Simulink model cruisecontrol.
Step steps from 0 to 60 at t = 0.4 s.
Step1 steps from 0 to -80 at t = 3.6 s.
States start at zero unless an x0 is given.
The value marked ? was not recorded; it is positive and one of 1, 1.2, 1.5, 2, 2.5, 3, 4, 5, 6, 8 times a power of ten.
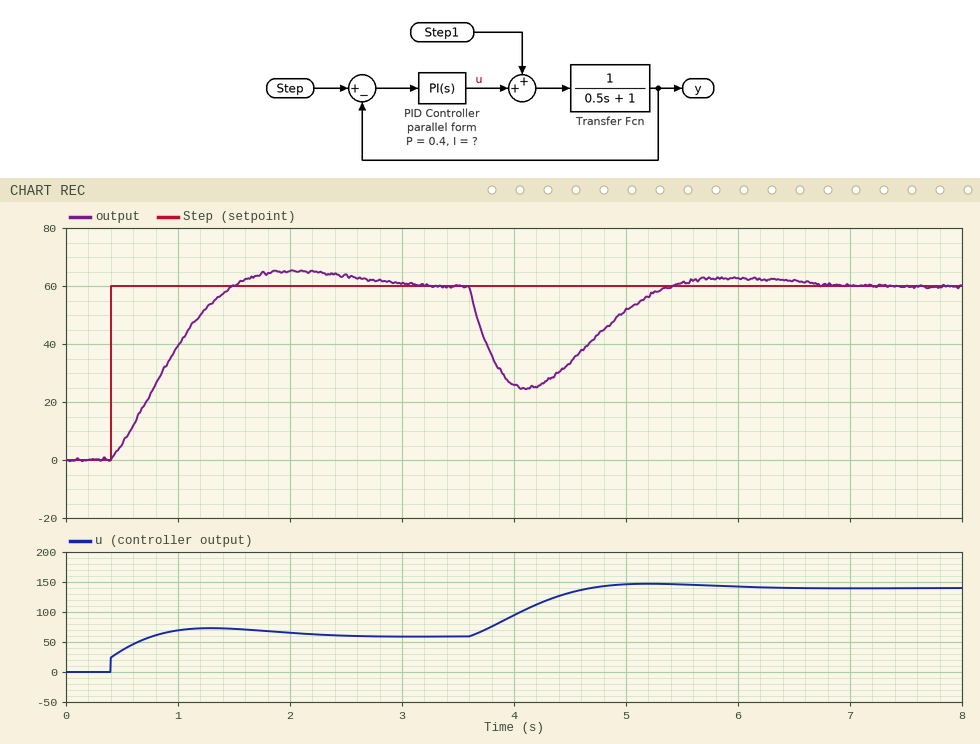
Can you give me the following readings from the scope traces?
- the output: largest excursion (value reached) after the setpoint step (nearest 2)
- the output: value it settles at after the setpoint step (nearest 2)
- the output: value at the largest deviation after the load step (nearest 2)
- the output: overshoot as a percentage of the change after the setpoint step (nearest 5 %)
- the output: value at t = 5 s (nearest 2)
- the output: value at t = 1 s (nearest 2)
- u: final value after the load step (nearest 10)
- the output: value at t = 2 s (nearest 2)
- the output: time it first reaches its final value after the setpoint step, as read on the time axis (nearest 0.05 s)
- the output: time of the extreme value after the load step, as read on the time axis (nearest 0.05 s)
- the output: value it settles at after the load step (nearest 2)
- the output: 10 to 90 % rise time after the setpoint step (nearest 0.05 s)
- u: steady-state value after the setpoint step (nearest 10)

66
60
24
10 %
52
40
140
66
1.50 s
4.10 s
60
0.80 s
60
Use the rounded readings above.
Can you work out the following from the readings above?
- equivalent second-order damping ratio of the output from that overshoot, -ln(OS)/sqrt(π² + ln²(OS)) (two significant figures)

0.59
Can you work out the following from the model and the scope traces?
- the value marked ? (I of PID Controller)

2.5
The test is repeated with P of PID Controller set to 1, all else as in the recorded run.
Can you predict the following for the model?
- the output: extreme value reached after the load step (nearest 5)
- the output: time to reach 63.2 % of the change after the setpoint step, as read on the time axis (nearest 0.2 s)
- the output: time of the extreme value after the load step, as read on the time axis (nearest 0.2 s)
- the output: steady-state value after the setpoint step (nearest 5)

30
0.8 s
4.0 s
60
